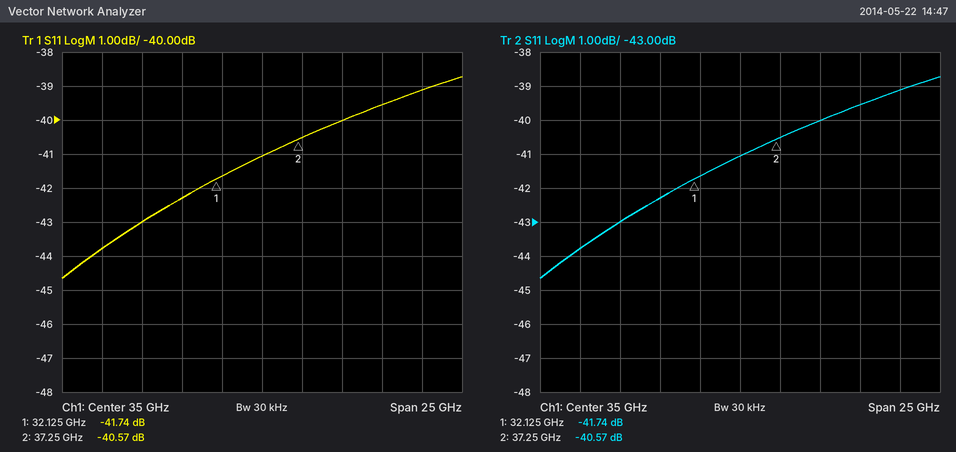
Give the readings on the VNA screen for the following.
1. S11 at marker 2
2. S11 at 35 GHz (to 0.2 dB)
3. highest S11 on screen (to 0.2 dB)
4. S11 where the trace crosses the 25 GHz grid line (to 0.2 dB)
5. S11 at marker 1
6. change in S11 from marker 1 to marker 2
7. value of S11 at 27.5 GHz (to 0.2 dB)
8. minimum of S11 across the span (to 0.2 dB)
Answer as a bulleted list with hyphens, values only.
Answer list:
- -40.57 dB
- -41.0 dB
- -38.8 dB
- -43.8 dB
- -41.74 dB
- 1.17 dB
- -43.0 dB
- -44.6 dB
